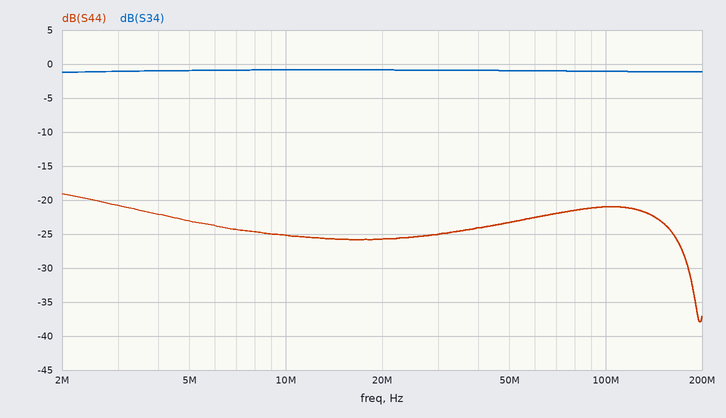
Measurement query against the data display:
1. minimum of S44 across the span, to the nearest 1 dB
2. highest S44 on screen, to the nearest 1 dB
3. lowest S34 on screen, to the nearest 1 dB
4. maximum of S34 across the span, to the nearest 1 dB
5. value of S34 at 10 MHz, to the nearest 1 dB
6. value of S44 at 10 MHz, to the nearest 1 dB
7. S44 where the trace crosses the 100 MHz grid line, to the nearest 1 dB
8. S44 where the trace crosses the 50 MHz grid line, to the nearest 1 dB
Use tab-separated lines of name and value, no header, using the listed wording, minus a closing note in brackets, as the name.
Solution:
minimum of S44 across the span, to the nearest 1 dB	-38 dB
highest S44 on screen, to the nearest 1 dB	-19 dB
lowest S34 on screen, to the nearest 1 dB	-1 dB
maximum of S34 across the span, to the nearest 1 dB	-1 dB
value of S34 at 10 MHz, to the nearest 1 dB	-1 dB
value of S44 at 10 MHz, to the nearest 1 dB	-25 dB
S44 where the trace crosses the 100 MHz grid line, to the nearest 1 dB	-21 dB
S44 where the trace crosses the 50 MHz grid line, to the nearest 1 dB	-23 dB
